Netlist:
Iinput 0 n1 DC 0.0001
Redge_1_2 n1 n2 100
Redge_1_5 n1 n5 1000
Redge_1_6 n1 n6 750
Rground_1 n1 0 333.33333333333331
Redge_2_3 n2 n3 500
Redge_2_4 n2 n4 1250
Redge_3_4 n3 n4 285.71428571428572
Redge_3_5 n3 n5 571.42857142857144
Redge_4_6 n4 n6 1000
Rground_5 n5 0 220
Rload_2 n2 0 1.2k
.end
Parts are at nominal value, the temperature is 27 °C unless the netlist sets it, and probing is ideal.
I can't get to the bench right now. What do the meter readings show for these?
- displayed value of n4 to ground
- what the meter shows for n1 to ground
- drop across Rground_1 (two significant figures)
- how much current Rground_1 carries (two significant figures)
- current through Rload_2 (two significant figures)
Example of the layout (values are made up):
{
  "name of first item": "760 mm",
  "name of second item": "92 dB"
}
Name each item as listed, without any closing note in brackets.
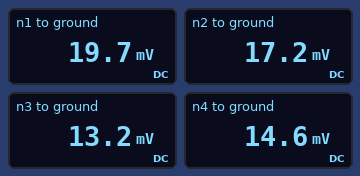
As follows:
{
  "displayed value of n4 to ground": "14.6 mV",
  "what the meter shows for n1 to ground": "19.7 mV",
  "drop across Rground_1": "20 mV",
  "how much current Rground_1 carries": "59 µA",
  "current through Rload_2": "14 µA"
}
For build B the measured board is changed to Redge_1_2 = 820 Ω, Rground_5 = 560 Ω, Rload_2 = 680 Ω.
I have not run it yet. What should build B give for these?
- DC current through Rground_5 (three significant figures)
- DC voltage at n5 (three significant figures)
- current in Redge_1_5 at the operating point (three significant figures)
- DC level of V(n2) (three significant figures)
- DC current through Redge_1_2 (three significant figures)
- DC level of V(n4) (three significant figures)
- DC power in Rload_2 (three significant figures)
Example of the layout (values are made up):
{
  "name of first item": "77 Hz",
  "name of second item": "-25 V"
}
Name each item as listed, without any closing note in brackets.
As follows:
{
  "DC current through Rground_5": "16.6 µA",
  "DC voltage at n5": "9.32 mV",
  "current in Redge_1_5 at the operating point": "13.1 µA",
  "DC level of V(n2)": "10.9 mV",
  "DC current through Redge_1_2": "14.0 µA",
  "DC level of V(n4)": "12.6 mV",
  "DC power in Rload_2": "176 nW"
}
